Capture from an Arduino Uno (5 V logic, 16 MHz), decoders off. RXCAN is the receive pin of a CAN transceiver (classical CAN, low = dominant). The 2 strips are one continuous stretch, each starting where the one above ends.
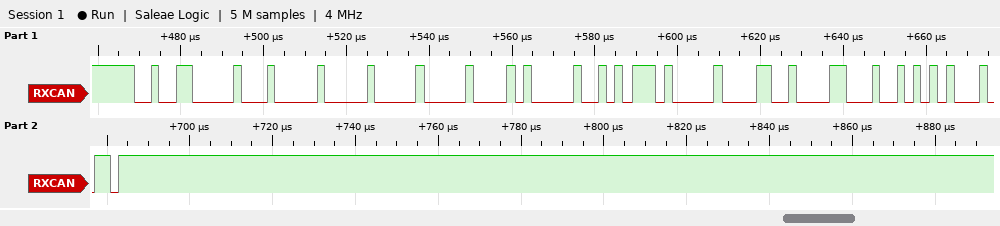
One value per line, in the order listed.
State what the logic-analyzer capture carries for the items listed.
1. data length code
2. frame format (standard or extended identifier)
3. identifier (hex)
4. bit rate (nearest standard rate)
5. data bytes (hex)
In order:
8
standard
0x260
500 kbit/s
00 00 05 01 5D 00 64 31
